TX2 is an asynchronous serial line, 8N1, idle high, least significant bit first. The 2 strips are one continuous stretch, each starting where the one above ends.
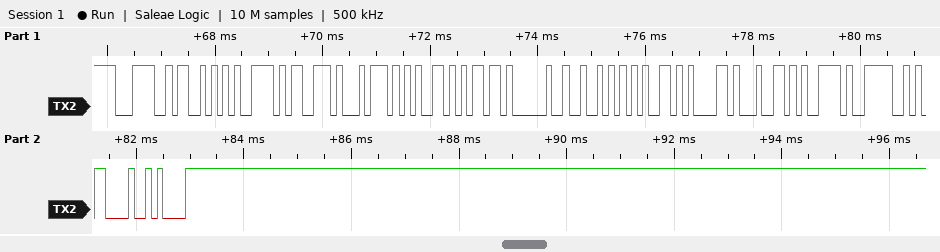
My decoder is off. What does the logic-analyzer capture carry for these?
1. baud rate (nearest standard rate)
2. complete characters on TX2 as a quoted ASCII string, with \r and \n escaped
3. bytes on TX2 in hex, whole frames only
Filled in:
9600 baud
"<System Ready>\r\n"
3C 53 79 73 74 65 6D 20 52 65 61 64 79 3E 0D 0A
